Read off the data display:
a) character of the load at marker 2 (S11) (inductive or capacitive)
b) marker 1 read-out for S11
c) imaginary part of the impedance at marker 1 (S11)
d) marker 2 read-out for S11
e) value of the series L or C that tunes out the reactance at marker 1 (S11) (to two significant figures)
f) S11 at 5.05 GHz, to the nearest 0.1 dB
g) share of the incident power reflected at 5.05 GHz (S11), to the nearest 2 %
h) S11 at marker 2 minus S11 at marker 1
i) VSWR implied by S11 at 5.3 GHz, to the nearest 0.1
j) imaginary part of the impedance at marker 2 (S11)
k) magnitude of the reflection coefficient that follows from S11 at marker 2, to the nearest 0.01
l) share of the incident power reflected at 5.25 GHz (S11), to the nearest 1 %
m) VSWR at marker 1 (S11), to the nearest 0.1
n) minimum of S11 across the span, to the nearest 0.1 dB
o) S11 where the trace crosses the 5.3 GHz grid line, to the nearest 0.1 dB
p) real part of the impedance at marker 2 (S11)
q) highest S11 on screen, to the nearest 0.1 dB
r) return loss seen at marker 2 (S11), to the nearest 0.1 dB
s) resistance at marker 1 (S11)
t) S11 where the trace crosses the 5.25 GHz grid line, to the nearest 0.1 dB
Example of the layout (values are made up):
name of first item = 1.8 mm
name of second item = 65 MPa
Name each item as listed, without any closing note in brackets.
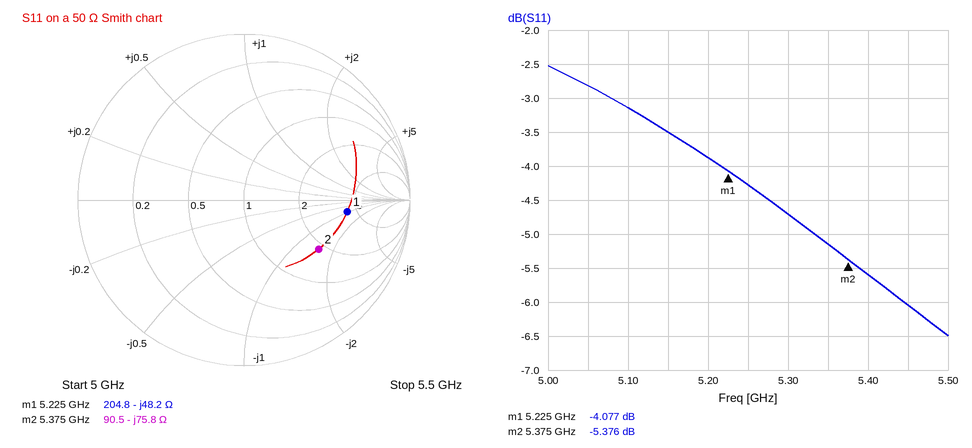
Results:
character of the load at marker 2 (S11) = capacitive
marker 1 read-out for S11 = -4.077 dB
imaginary part of the impedance at marker 1 = -48.2 Ω
marker 2 read-out for S11 = -5.376 dB
value of the series L or C that tunes out the reactance at marker 1 (S11) = 1.5 nH
S11 at 5.05 GHz, to the nearest 0.1 dB = -2.8 dB
share of the incident power reflected at 5.05 GHz (S11), to the nearest 2 % = 52 %
S11 at marker 2 minus S11 at marker 1 = -1.299 dB
VSWR implied by S11 at 5.3 GHz, to the nearest 0.1 = 3.8
imaginary part of the impedance at marker 2 = -75.8 Ω
magnitude of the reflection coefficient that follows from S11 at marker 2, to the nearest 0.01 = 0.54
share of the incident power reflected at 5.25 GHz (S11), to the nearest 1 % = 37 %
VSWR at marker 1 (S11), to the nearest 0.1 = 4.3
minimum of S11 across the span, to the nearest 0.1 dB = -6.5 dB
S11 where the trace crosses the 5.3 GHz grid line, to the nearest 0.1 dB = -4.7 dB
real part of the impedance at marker 2 = 90.5 Ω
highest S11 on screen, to the nearest 0.1 dB = -2.5 dB
return loss seen at marker 2 (S11), to the nearest 0.1 dB = 5.4 dB
resistance at marker 1 = 204.8 Ω
S11 where the trace crosses the 5.25 GHz grid line, to the nearest 0.1 dB = -4.3 dB
